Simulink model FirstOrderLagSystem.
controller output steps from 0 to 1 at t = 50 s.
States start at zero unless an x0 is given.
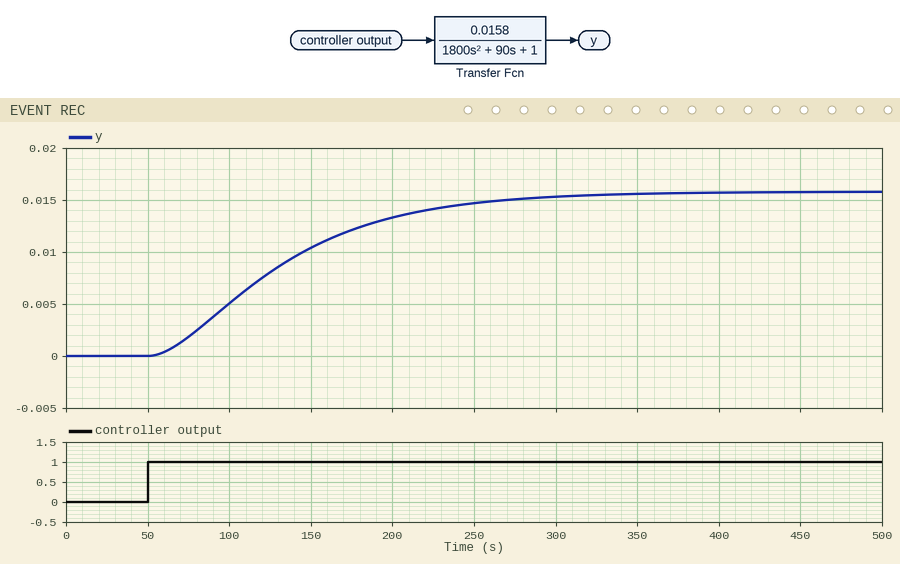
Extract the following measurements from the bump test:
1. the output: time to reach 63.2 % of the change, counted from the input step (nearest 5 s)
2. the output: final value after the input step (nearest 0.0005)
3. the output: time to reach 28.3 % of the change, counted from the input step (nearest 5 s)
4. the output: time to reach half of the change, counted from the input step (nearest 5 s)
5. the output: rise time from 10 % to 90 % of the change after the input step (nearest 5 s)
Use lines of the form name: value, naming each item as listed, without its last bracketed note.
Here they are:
the output: time to reach 63.2 % of the change, counted from the input step: 95 s
the output: final value after the input step: 0.0160
the output: time to reach 28.3 % of the change, counted from the input step: 45 s
the output: time to reach half of the change, counted from the input step: 75 s
the output: rise time from 10 % to 90 % of the change after the input step: 155 s
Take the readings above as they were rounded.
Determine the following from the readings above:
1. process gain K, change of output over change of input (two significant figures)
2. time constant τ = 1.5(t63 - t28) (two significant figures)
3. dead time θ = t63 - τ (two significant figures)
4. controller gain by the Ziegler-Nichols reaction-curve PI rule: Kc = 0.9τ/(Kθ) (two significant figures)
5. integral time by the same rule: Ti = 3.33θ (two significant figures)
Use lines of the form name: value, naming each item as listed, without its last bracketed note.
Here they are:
process gain K, change of output over change of input: 0.016
time constant τ = 1.5(t63 - t28): 75 s
dead time θ = t63 - τ: 20 s
controller gain by the Ziegler-Nichols reaction-curve PI rule: Kc = 0.9τ/(Kθ): 210
integral time by the same rule: Ti = 3.33θ: 67 s
